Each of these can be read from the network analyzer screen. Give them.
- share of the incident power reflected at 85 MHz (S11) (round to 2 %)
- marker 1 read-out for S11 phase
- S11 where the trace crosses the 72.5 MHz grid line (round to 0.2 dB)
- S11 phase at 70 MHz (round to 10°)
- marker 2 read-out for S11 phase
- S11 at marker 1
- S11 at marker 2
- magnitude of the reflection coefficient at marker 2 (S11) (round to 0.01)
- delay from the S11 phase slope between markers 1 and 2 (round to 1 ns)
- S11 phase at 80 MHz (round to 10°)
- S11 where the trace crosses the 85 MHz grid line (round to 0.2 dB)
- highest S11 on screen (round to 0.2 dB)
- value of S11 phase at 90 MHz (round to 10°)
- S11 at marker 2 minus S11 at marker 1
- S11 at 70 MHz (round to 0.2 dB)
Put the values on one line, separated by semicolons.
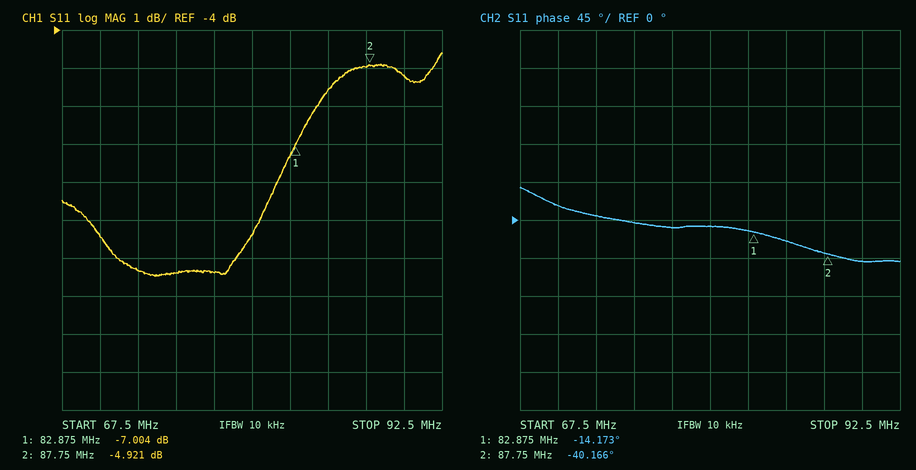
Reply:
28 %; -14.173°; -10.4 dB; 20°; -40.166°; -7.004 dB; -4.921 dB; 0.57; 15 ns; -10°; -5.6 dB; -4.6 dB; -50°; 2.083 dB; -9.4 dB
